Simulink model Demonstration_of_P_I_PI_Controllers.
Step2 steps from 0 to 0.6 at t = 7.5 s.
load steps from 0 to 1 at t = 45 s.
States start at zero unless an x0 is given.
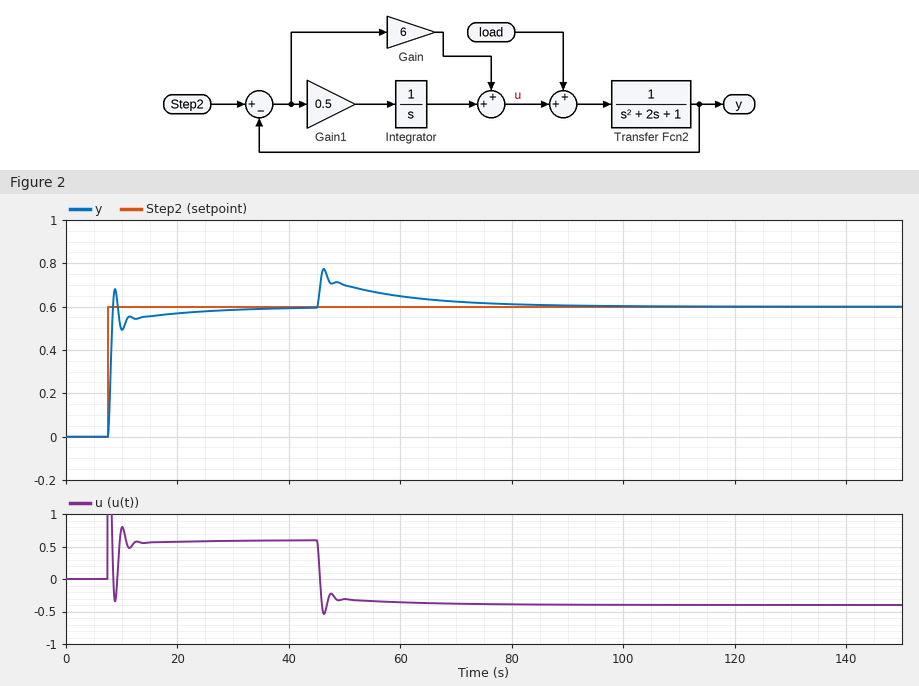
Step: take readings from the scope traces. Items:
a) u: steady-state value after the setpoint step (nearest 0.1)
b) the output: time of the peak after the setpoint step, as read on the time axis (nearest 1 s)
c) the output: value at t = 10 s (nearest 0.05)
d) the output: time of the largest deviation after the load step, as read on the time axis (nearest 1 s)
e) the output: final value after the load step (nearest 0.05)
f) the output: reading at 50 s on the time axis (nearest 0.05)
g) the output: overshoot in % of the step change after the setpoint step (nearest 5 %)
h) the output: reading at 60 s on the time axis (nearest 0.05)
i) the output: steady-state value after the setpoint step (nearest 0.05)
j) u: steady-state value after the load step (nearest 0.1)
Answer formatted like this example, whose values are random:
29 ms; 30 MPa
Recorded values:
0.6; 9 s; 0.50; 46 s; 0.60; 0.70; 15 %; 0.65; 0.60; -0.4
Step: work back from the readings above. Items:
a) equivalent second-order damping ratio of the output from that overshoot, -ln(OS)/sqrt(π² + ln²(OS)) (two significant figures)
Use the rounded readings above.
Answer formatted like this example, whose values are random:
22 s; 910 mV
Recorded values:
0.52
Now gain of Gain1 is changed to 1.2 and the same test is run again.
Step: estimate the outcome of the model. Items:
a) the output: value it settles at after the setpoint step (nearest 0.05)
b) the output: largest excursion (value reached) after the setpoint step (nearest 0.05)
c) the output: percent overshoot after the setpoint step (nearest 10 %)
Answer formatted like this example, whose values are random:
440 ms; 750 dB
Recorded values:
0.60; 0.70; 20 %
